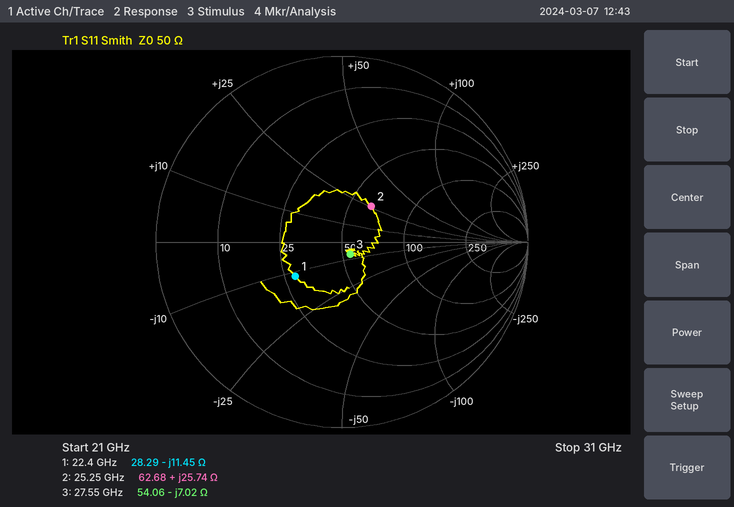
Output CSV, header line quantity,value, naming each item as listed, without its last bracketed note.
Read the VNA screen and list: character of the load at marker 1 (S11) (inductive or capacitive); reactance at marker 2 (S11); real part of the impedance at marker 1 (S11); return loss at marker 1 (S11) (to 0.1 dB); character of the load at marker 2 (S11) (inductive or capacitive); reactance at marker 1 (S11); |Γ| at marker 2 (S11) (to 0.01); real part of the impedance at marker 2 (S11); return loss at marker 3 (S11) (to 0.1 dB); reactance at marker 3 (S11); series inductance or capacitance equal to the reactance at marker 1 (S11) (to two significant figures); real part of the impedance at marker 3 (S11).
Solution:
quantity,value
character of the load at marker 1 (S11),capacitive
reactance at marker 2,+25.74 Ω
real part of the impedance at marker 1,28.29 Ω
return loss at marker 1 (S11),10.2 dB
character of the load at marker 2 (S11),inductive
reactance at marker 1,-11.45 Ω
|Γ| at marker 2 (S11),0.25
real part of the impedance at marker 2,62.68 Ω
return loss at marker 3 (S11),22.2 dB
reactance at marker 3,-7.02 Ω
series inductance or capacitance equal to the reactance at marker 1 (S11),620 fF
real part of the impedance at marker 3,54.06 Ω
